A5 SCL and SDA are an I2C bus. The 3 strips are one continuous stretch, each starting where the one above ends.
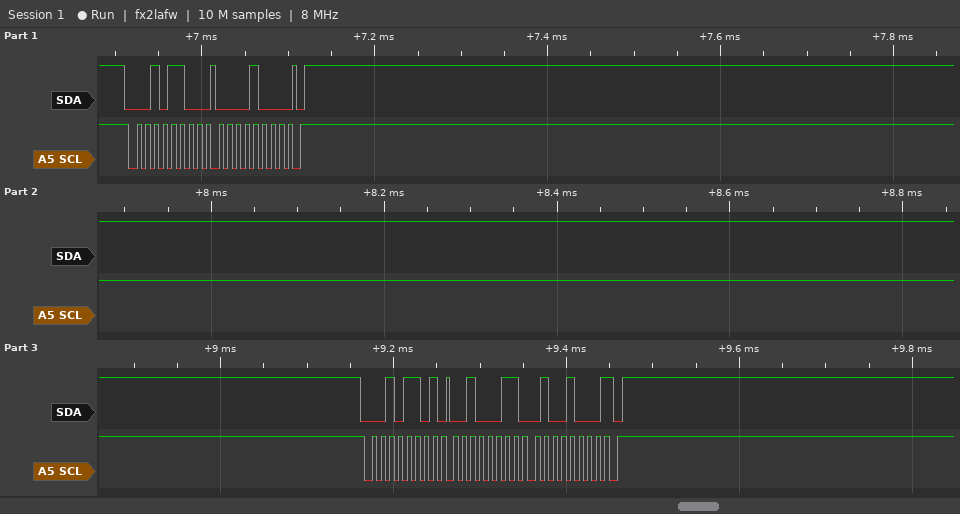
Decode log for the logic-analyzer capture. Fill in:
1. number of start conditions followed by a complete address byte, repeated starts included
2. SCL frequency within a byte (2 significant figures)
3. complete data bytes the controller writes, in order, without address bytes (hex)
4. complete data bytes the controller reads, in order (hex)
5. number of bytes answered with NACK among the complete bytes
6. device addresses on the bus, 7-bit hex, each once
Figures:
2
100 kHz
08
23 48
1
0x16
